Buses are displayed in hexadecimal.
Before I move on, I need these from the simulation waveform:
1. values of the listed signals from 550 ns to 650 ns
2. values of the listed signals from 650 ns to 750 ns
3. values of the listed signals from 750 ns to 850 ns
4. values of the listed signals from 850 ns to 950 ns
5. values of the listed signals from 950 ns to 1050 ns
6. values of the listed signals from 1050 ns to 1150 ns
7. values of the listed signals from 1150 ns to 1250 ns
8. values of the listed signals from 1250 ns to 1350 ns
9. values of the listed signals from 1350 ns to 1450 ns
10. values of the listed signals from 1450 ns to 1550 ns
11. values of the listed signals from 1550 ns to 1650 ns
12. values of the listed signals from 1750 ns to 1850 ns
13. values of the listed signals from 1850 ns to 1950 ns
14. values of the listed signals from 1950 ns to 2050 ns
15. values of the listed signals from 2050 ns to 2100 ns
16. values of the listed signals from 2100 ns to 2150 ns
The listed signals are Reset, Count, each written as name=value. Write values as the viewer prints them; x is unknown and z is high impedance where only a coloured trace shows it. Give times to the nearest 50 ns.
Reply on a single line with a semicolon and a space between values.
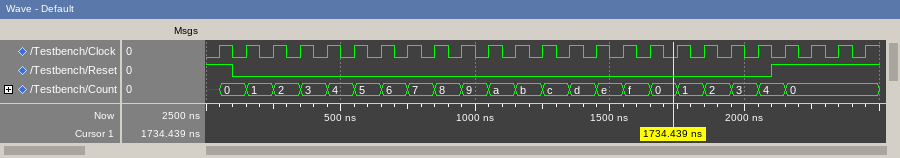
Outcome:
Reset=0, Count=5; Reset=0, Count=6; Reset=0, Count=7; Reset=0, Count=8; Reset=0, Count=9; Reset=0, Count=a; Reset=0, Count=b; Reset=0, Count=c; Reset=0, Count=d; Reset=0, Count=e; Reset=0, Count=f; Reset=0, Count=1; Reset=0, Count=2; Reset=0, Count=3; Reset=0, Count=4; Reset=1, Count=4
